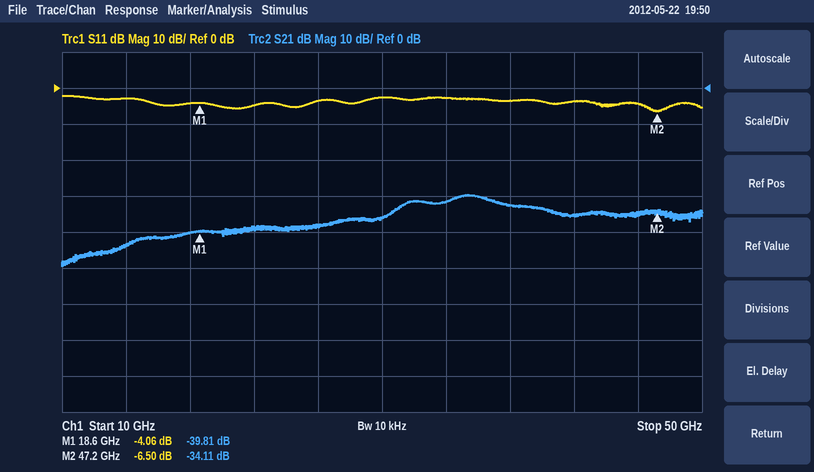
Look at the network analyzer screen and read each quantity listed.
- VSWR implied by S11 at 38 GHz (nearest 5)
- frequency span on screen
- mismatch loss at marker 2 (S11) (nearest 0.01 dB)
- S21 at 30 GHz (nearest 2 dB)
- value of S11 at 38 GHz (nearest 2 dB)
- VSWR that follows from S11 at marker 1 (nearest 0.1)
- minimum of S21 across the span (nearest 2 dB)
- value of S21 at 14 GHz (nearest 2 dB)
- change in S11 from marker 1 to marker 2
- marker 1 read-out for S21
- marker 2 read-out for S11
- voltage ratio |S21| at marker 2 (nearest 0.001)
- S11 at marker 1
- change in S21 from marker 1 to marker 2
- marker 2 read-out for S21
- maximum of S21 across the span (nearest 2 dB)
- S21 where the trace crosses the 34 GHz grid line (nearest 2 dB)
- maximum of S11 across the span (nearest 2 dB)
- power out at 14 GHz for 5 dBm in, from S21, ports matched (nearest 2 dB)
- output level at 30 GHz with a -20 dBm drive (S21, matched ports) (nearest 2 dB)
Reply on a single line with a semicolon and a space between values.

5; 40 GHz; 1.10 dB; -36 dB; -4 dB; 4.4; -50 dB; -44 dB; -2.44 dB; -39.81 dB; -6.50 dB; 0.020; -4.06 dB; 5.70 dB; -34.11 dB; -30 dB; -32 dB; -2 dB; -38 dBm; -56 dBm
